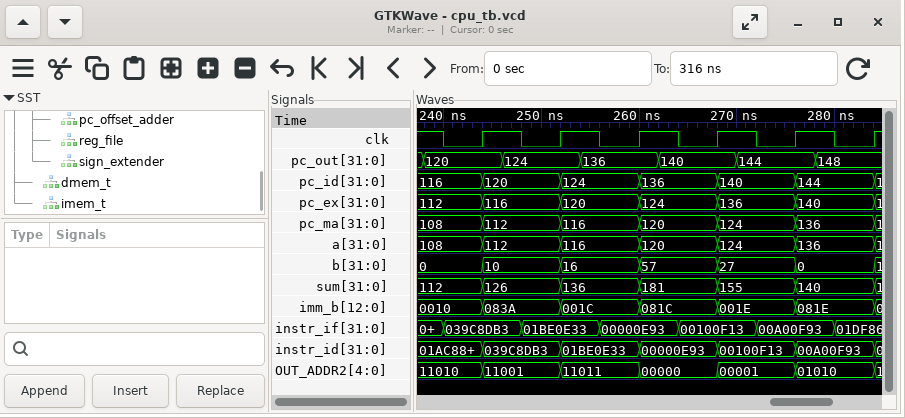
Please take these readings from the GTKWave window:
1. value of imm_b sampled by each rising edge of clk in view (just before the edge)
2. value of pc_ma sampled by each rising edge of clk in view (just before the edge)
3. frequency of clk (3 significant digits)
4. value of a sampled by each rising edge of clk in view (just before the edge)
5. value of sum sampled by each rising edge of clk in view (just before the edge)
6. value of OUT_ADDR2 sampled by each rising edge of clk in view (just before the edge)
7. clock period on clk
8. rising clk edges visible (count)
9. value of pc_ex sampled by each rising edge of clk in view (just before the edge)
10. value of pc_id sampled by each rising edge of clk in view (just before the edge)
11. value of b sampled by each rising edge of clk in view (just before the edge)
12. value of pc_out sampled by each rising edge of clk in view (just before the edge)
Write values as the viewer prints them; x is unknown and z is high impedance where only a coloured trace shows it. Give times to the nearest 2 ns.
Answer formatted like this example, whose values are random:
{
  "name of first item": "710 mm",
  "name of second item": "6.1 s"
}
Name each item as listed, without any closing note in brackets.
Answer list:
{
  "value of imm_b sampled by each rising edge of clk in view": "0010, 083A, 001C, 081C, 001E, 081E",
  "value of pc_ma sampled by each rising edge of clk in view": "108, 112, 116, 120, 124, 136",
  "frequency of clk": "125 MHz",
  "value of a sampled by each rising edge of clk in view": "108, 112, 116, 120, 124, 136",
  "value of sum sampled by each rising edge of clk in view": "112, 126, 136, 181, 155, 140",
  "value of OUT_ADDR2 sampled by each rising edge of clk in view": "11010, 11001, 11011, 00000, 00001, 01010",
  "clock period on clk": "8 ns",
  "rising clk edges visible": "6",
  "value of pc_ex sampled by each rising edge of clk in view": "112, 116, 120, 124, 136, 140",
  "value of pc_id sampled by each rising edge of clk in view": "116, 120, 124, 136, 140, 144",
  "value of b sampled by each rising edge of clk in view": "0, 10, 16, 57, 27, 0",
  "value of pc_out sampled by each rising edge of clk in view": "120, 124, 136, 140, 144, 148"
}
